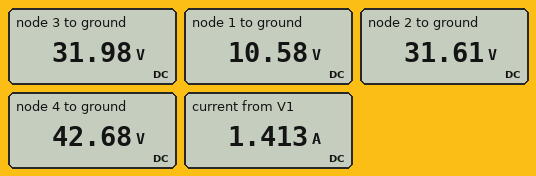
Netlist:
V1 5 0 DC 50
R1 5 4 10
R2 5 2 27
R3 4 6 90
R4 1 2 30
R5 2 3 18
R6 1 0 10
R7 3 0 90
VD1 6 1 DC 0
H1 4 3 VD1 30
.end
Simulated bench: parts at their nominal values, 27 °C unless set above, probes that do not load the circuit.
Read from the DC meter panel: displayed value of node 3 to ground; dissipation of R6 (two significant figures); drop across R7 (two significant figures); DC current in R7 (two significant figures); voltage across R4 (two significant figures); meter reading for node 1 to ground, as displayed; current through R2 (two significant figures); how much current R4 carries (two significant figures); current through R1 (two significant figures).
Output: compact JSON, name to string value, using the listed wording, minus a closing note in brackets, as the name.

{"displayed value of node 3 to ground": "31.98 V", "dissipation of R6": "11 W", "drop across R7": "32 V", "DC current in R7": "360 mA", "voltage across R4": "21 V", "meter reading for node 1 to ground, as displayed": "10.58 V", "current through R2": "680 mA", "how much current R4 carries": "700 mA", "current through R1": "730 mA"}
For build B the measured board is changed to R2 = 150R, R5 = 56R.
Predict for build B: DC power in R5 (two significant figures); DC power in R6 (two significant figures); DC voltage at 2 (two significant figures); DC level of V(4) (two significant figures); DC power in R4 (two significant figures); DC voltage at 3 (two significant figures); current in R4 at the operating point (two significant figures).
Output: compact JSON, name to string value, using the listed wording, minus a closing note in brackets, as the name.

{"DC power in R5": "2.0 W", "DC power in R6": "5.8 W", "DC voltage at 2": "19 V", "DC level of V(4)": "41 V", "DC power in R4": "4.6 W", "DC voltage at 3": "30 V", "current in R4 at the operating point": "390 mA"}
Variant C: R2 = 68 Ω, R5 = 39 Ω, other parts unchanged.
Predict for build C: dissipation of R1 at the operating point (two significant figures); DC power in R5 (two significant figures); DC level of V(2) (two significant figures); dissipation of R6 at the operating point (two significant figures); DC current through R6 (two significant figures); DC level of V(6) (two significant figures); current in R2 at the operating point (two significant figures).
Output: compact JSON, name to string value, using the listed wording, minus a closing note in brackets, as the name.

{"dissipation of R1 at the operating point": "7.3 W", "DC power in R5": "910 mW", "DC level of V(2)": "25 V", "dissipation of R6 at the operating point": "7.9 W", "DC current through R6": "890 mA", "DC level of V(6)": "8.9 V", "current in R2 at the operating point": "370 mA"}
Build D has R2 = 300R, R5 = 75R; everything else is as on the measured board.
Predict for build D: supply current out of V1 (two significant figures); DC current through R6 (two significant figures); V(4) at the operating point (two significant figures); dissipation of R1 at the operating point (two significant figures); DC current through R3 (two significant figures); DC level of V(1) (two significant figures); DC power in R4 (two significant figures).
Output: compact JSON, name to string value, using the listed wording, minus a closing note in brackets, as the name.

{"supply current out of V1": "1.0 A", "DC current through R6": "680 mA", "V(4) at the operating point": "41 V", "dissipation of R1 at the operating point": "8.0 W", "DC current through R3": "380 mA", "DC level of V(1)": "6.8 V", "DC power in R4": "2.7 W"}
